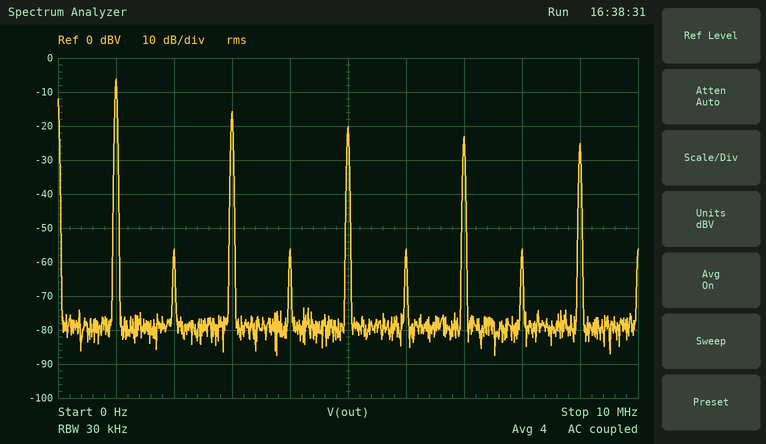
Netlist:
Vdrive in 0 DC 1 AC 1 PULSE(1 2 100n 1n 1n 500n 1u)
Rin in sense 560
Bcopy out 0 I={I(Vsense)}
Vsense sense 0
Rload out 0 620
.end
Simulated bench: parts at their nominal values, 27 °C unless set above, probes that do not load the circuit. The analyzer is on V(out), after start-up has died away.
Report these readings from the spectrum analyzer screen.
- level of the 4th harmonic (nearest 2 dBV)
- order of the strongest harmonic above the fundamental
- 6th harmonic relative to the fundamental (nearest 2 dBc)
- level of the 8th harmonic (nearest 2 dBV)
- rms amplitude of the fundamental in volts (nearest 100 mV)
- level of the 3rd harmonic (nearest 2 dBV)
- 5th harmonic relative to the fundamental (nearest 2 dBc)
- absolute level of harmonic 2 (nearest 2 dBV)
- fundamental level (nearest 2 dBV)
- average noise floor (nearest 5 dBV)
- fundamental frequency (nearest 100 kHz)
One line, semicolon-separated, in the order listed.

-56 dBV; 3; -50 dBc; -56 dBV; 500 mV; -16 dBV; -14 dBc; -56 dBV; -6 dBV; -80 dBV; 1.0 MHz
